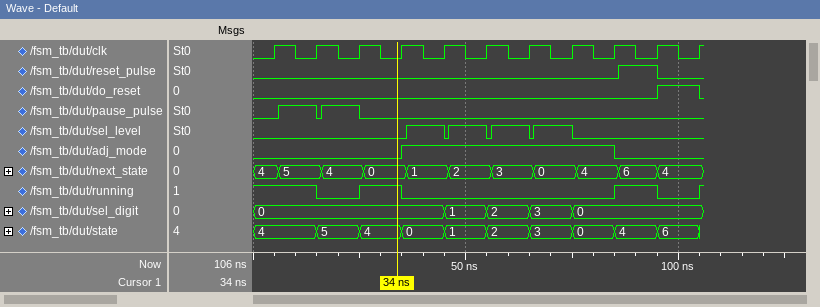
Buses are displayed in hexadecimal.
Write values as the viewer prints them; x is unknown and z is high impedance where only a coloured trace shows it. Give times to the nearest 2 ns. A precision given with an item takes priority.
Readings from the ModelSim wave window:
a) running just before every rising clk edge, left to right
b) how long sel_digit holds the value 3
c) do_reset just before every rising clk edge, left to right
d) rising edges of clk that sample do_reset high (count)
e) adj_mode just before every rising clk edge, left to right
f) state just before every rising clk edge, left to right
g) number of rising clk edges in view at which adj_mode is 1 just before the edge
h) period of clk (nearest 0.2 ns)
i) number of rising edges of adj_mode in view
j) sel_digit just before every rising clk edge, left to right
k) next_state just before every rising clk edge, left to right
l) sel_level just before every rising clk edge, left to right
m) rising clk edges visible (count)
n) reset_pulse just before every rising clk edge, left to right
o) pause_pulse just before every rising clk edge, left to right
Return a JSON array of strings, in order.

["1 1 0 1 0 0 0 0 0 1 0", "10 ns", "0 0 0 0 0 0 0 0 0 0 1", "1", "0 0 0 0 1 1 1 1 1 0 0", "4, 4, 5, 4, 0, 1, 2, 3, 0, 4, 6", "5", "10 ns", "1", "0, 0, 0, 0, 0, 1, 2, 3, 0, 0, 0", "4, 5, 4, 0, 1, 2, 3, 0, 4, 6, 4", "0 0 0 0 1 1 1 1 0 0 0", "11", "0 0 0 0 0 0 0 0 0 1 0", "0 1 1 0 0 0 0 0 0 0 0"]
